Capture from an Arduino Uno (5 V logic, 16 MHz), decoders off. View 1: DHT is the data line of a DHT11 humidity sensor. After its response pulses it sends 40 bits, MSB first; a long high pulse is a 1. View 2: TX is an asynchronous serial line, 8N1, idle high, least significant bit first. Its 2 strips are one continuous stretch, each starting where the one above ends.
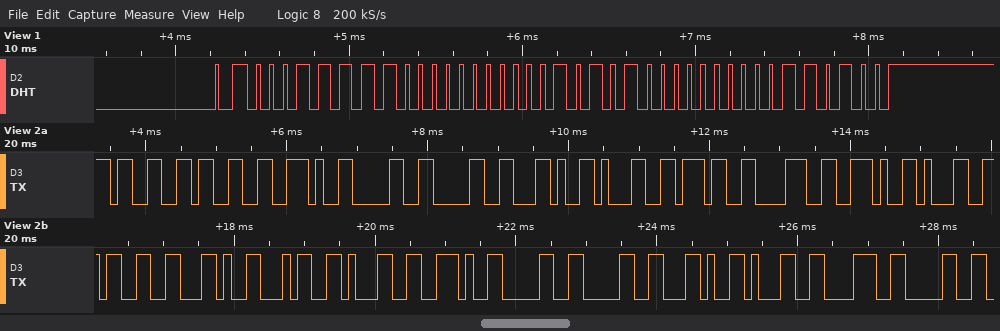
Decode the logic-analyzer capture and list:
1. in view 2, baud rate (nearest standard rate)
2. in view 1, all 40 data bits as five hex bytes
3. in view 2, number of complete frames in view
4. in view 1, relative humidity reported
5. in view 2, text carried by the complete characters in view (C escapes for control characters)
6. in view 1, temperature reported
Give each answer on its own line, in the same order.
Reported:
9600 baud
1F 00 15 00 34
22
31 %
"33.00,178.13,41.00,180"
21.0 °C
